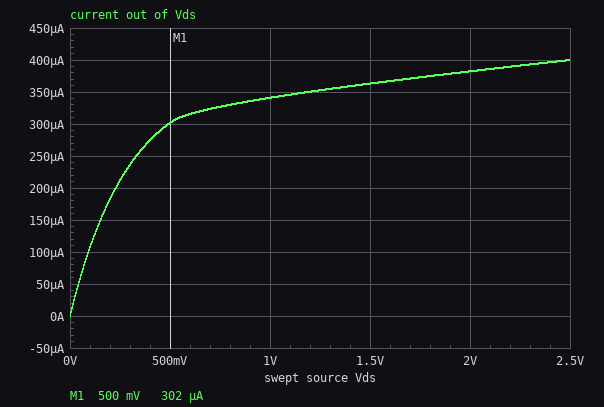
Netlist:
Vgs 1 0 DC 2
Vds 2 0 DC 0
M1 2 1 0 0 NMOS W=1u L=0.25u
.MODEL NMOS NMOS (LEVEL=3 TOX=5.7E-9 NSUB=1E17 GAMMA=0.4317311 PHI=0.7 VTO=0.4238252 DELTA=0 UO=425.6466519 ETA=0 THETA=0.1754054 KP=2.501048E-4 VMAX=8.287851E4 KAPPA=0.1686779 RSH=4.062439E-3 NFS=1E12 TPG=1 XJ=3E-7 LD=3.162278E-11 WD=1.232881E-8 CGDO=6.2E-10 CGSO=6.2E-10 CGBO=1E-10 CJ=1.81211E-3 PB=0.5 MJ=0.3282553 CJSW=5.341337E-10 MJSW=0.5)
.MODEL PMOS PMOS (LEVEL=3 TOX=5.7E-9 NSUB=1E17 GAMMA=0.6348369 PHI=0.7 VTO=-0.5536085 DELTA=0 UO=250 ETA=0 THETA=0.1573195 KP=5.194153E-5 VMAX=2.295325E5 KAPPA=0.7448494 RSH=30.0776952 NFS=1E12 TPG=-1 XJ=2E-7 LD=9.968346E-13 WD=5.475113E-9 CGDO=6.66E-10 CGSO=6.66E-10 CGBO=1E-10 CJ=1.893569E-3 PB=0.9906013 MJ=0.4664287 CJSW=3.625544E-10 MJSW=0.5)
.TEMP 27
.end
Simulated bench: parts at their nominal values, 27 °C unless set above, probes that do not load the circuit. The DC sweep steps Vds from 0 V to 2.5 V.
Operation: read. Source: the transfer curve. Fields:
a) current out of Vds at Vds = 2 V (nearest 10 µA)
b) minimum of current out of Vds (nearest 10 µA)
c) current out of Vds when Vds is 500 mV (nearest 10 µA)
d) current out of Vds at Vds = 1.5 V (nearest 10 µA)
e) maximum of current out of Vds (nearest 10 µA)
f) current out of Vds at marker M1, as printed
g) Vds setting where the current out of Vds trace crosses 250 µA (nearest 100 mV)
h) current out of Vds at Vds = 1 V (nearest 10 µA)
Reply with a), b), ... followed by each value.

a) 380 µA
b) 0 A
c) 300 µA
d) 360 µA
e) 400 µA
f) 302 µA
g) 300 mV
h) 340 µA
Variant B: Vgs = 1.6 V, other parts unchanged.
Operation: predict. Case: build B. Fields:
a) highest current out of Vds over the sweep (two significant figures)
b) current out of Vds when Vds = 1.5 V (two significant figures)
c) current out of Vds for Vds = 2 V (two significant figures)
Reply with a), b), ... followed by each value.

a) 290 µA
b) 260 µA
c) 280 µA
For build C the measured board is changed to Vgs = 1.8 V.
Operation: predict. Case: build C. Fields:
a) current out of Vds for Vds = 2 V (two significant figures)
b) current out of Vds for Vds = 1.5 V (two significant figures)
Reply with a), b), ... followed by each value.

a) 330 µA
b) 310 µA
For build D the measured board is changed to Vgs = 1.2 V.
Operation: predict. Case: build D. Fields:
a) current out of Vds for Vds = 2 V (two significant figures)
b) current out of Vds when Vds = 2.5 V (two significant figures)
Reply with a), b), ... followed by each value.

a) 170 µA
b) 180 µA
